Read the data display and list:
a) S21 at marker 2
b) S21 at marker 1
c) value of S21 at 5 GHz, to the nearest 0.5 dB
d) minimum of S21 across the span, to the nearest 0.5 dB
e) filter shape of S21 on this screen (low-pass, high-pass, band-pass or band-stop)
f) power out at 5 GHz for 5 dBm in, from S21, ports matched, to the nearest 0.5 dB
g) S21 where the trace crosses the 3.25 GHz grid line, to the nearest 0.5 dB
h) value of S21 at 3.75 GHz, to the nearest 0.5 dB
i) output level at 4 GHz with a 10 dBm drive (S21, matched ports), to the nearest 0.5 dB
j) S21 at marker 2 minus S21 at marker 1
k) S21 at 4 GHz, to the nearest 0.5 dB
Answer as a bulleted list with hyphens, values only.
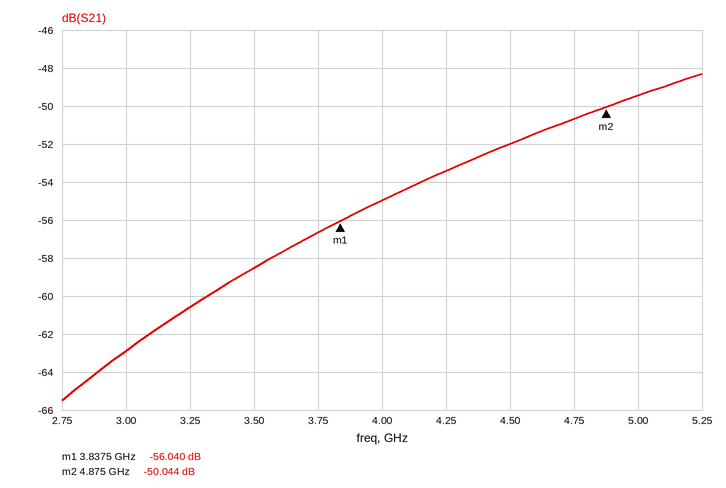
- -50.044 dB
- -56.040 dB
- -49.5 dB
- -65.5 dB
- high-pass
- -44.5 dBm
- -60.5 dB
- -56.5 dB
- -45.0 dBm
- 5.996 dB
- -55.0 dB
